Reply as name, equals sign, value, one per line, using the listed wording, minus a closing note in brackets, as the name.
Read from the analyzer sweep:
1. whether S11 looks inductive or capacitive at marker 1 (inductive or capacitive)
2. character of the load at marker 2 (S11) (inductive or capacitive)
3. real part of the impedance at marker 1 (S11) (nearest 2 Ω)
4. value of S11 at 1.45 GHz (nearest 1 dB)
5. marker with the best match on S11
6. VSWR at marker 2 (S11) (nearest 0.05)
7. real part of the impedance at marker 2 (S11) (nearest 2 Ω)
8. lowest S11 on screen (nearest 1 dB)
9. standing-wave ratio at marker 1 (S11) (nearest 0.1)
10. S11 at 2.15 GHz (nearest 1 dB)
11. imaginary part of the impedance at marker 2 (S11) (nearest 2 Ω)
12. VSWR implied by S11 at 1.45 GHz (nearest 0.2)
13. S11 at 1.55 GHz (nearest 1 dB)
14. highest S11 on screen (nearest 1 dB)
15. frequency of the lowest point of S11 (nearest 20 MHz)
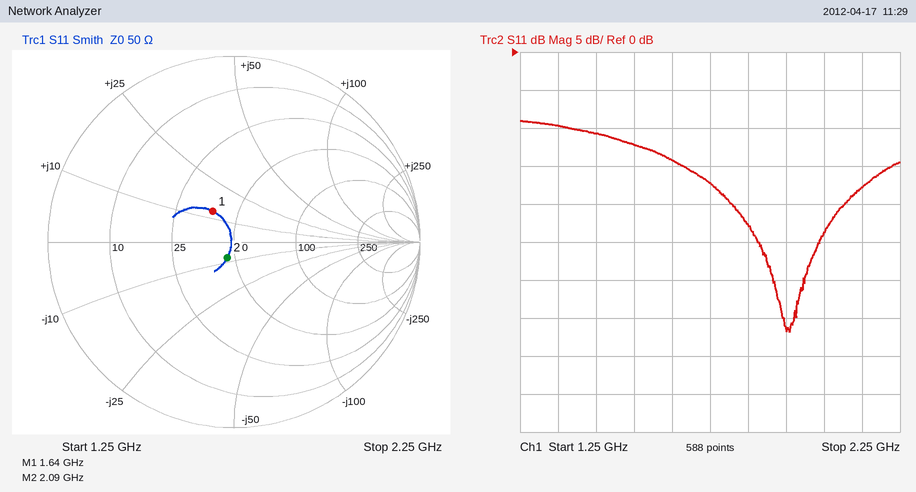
whether S11 looks inductive or capacitive at marker 1 = inductive
character of the load at marker 2 (S11) = capacitive
real part of the impedance at marker 1 (S11) = 38 Ω
value of S11 at 1.45 GHz = -11 dB
marker with the best match on S11 = marker 2
VSWR at marker 2 (S11) = 1.20
real part of the impedance at marker 2 (S11) = 46 Ω
lowest S11 on screen = -37 dB
standing-wave ratio at marker 1 (S11) = 1.5
S11 at 2.15 GHz = -18 dB
imaginary part of the impedance at marker 2 (S11) = -8 Ω
VSWR implied by S11 at 1.45 GHz = 1.8
S11 at 1.55 GHz = -12 dB
highest S11 on screen = -9 dB
frequency of the lowest point of S11 = 1.96 GHz
